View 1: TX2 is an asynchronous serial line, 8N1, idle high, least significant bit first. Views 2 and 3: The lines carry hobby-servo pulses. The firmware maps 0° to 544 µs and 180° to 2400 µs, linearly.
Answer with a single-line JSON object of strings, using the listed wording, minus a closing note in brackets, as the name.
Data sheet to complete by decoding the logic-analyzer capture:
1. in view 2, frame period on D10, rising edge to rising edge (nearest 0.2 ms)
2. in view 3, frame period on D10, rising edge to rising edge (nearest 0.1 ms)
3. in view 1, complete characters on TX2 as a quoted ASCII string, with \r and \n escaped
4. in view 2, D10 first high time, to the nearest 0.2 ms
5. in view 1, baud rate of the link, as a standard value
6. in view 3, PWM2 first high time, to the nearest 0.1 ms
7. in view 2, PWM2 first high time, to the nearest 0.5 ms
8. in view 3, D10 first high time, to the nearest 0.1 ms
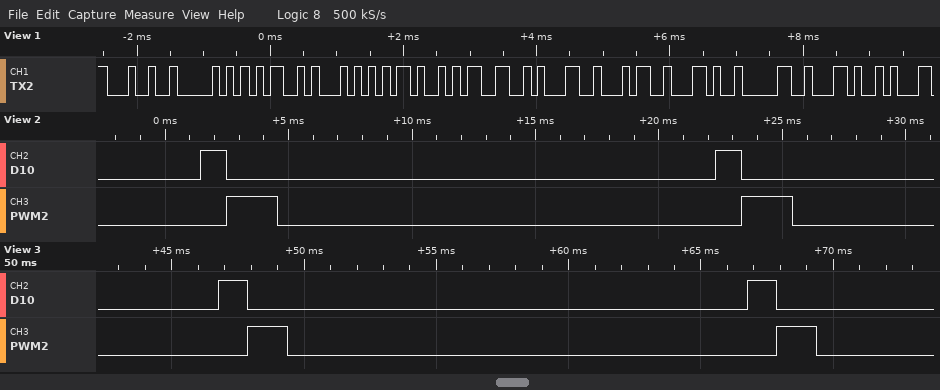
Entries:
{"in view 2, frame period on D10, rising edge to rising edge": "20.8 ms", "in view 3, frame period on D10, rising edge to rising edge": "20.0 ms", "in view 1, complete characters on TX2 as a quoted ASCII string, with \\r and \\n escaped": "\"$PMTK314,0,\"", "in view 2, D10 first high time, to the nearest 0.2 ms": "1.0 ms", "in view 1, baud rate of the link, as a standard value": "9600 baud", "in view 3, PWM2 first high time, to the nearest 0.1 ms": "1.5 ms", "in view 2, PWM2 first high time, to the nearest 0.5 ms": "2.0 ms", "in view 3, D10 first high time, to the nearest 0.1 ms": "1.1 ms"}
